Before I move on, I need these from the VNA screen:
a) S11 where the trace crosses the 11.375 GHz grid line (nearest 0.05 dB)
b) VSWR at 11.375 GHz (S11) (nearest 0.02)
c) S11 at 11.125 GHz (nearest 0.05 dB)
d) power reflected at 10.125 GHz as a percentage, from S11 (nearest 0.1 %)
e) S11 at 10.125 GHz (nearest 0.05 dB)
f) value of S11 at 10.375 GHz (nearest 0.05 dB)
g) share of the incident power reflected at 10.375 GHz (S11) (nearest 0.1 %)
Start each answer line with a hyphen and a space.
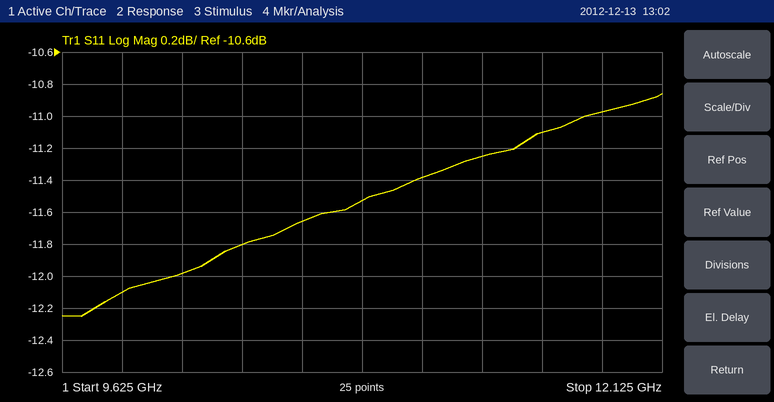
- -11.25 dB
- 1.76
- -11.40 dB
- 6.3 %
- -12.00 dB
- -11.80 dB
- 6.6 %
